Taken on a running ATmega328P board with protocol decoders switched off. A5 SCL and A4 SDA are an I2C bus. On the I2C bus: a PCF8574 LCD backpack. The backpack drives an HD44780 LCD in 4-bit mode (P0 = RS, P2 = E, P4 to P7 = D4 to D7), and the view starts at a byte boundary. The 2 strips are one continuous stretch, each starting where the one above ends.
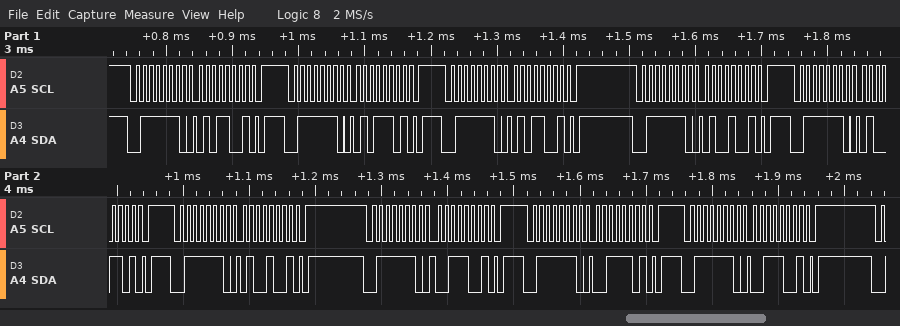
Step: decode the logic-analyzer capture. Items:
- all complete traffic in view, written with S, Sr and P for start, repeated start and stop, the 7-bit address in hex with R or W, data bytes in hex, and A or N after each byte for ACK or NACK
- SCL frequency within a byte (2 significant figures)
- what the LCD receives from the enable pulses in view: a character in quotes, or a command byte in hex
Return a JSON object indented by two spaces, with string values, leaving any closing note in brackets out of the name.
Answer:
{
  "all complete traffic in view, written with S, Sr and P for start, repeated start and stop, the 7-bit address in hex with R or W, data bytes in hex, and A or N after each byte for ACK or NACK": "S 3FW A 59 A P S 3FW A 5D A P S 3FW A 59 A P S 3FW A 49 A P S 3FW A 4D A P S 3FW A 49 A P S 3FW A 39 A P S 3FW A 3D A P S 3FW A 39 A P",
  "SCL frequency within a byte": "100 kHz",
  "what the LCD receives from the enable pulses in view: a character in quotes, or a command byte in hex": "'T'"
}
